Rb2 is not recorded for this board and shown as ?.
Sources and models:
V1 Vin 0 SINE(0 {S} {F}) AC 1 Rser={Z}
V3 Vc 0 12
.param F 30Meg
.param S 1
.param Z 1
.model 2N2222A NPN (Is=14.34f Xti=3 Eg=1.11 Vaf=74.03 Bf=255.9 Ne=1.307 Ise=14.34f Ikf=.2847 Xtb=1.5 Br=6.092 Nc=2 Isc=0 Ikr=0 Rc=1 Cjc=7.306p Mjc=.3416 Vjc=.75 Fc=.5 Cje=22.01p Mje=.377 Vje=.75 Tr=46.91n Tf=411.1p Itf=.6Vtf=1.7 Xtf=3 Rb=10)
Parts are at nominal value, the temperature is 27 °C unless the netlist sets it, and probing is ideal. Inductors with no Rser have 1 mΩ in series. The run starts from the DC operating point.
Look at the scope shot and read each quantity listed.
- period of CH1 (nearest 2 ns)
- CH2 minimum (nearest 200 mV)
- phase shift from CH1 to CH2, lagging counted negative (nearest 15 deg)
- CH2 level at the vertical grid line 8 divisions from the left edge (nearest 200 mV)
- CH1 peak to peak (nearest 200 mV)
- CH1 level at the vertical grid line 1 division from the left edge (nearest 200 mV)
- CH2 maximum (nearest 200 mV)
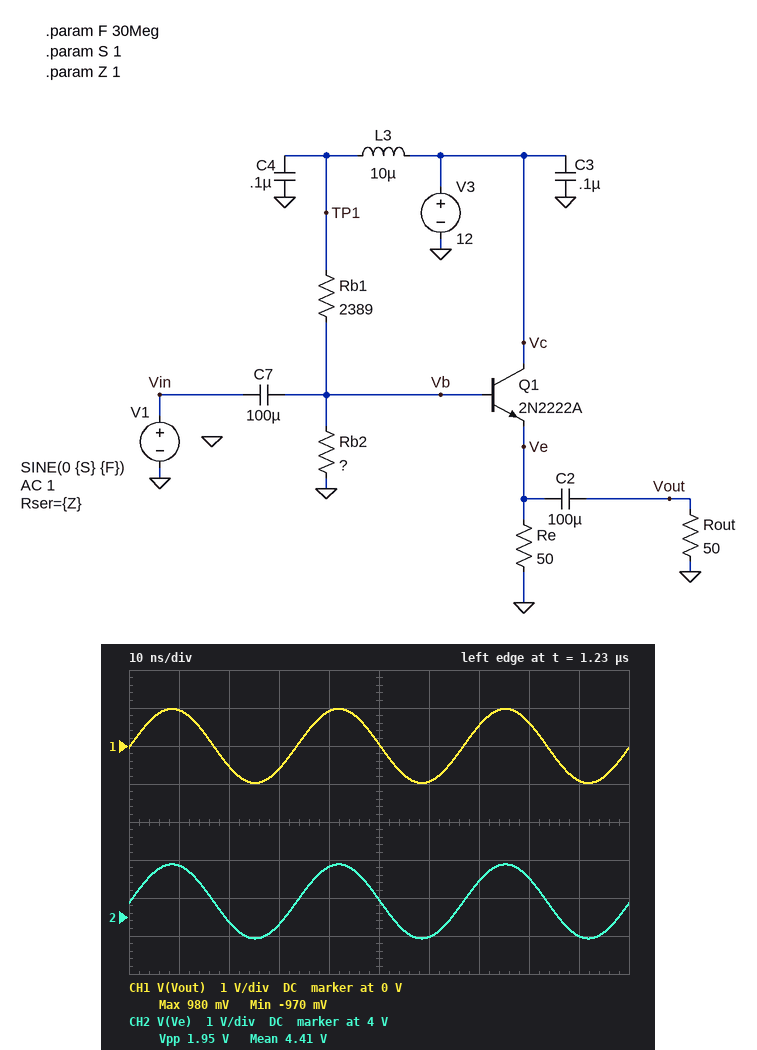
34 ns
3.4 V
0 deg
5.0 V
2.0 V
1.0 V
5.4 V
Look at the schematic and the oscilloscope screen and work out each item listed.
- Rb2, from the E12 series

2.2 kΩ
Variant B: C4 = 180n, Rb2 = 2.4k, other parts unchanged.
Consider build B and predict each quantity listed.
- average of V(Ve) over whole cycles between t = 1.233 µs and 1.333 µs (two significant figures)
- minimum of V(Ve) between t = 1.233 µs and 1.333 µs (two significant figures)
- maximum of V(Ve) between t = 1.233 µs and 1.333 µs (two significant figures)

4.6 V
3.6 V
5.6 V
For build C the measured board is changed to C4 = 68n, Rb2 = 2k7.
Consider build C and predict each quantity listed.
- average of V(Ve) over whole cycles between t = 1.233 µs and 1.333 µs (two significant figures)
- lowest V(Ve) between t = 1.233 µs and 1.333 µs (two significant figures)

4.9 V
3.9 V
